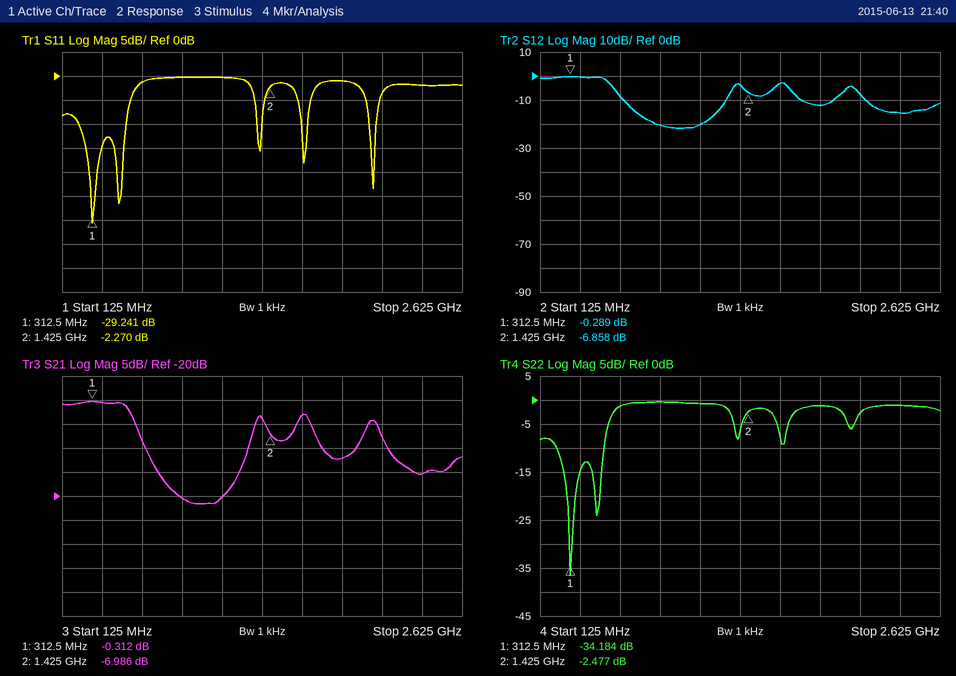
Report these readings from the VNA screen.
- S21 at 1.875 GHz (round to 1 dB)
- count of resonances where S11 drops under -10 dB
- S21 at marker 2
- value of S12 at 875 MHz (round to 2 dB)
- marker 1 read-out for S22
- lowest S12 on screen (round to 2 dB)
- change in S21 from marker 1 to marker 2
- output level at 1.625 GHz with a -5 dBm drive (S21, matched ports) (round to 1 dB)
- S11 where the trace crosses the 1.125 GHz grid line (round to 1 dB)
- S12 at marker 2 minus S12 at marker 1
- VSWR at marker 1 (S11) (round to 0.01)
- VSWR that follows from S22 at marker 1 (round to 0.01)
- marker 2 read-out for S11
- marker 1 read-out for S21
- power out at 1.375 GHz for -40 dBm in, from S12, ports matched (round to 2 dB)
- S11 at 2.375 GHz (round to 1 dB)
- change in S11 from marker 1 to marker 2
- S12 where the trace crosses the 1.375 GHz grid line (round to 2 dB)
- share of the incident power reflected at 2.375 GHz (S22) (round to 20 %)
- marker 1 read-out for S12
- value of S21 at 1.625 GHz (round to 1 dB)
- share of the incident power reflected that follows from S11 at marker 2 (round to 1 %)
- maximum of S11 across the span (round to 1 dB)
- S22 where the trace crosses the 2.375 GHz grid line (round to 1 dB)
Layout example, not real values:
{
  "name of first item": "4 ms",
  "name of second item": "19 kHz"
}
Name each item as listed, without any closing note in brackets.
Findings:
{
  "S21 at 1.875 GHz": "-12 dB",
  "count of resonances where S11 drops under -10 dB": "5",
  "S21 at marker 2": "-6.986 dB",
  "value of S12 at 875 MHz": "-20 dB",
  "marker 1 read-out for S22": "-34.184 dB",
  "lowest S12 on screen": "-22 dB",
  "change in S21 from marker 1 to marker 2": "-6.674 dB",
  "output level at 1.625 GHz with a -5 dBm drive (S21, matched ports)": "-8 dBm",
  "S11 where the trace crosses the 1.125 GHz grid line": "0 dB",
  "S12 at marker 2 minus S12 at marker 1": "-6.569 dB",
  "VSWR at marker 1 (S11)": "1.07",
  "VSWR that follows from S22 at marker 1": "1.04",
  "marker 2 read-out for S11": "-2.270 dB",
  "marker 1 read-out for S21": "-0.312 dB",
  "power out at 1.375 GHz for -40 dBm in, from S12, ports matched": "-44 dBm",
  "S11 at 2.375 GHz": "-2 dB",
  "change in S11 from marker 1 to marker 2": "26.971 dB",
  "S12 where the trace crosses the 1.375 GHz grid line": "-4 dB",
  "share of the incident power reflected at 2.375 GHz (S22)": "80 %",
  "marker 1 read-out for S12": "-0.289 dB",
  "value of S21 at 1.625 GHz": "-3 dB",
  "share of the incident power reflected that follows from S11 at marker 2": "59 %",
  "maximum of S11 across the span": "0 dB",
  "S22 where the trace crosses the 2.375 GHz grid line": "-1 dB"
}
